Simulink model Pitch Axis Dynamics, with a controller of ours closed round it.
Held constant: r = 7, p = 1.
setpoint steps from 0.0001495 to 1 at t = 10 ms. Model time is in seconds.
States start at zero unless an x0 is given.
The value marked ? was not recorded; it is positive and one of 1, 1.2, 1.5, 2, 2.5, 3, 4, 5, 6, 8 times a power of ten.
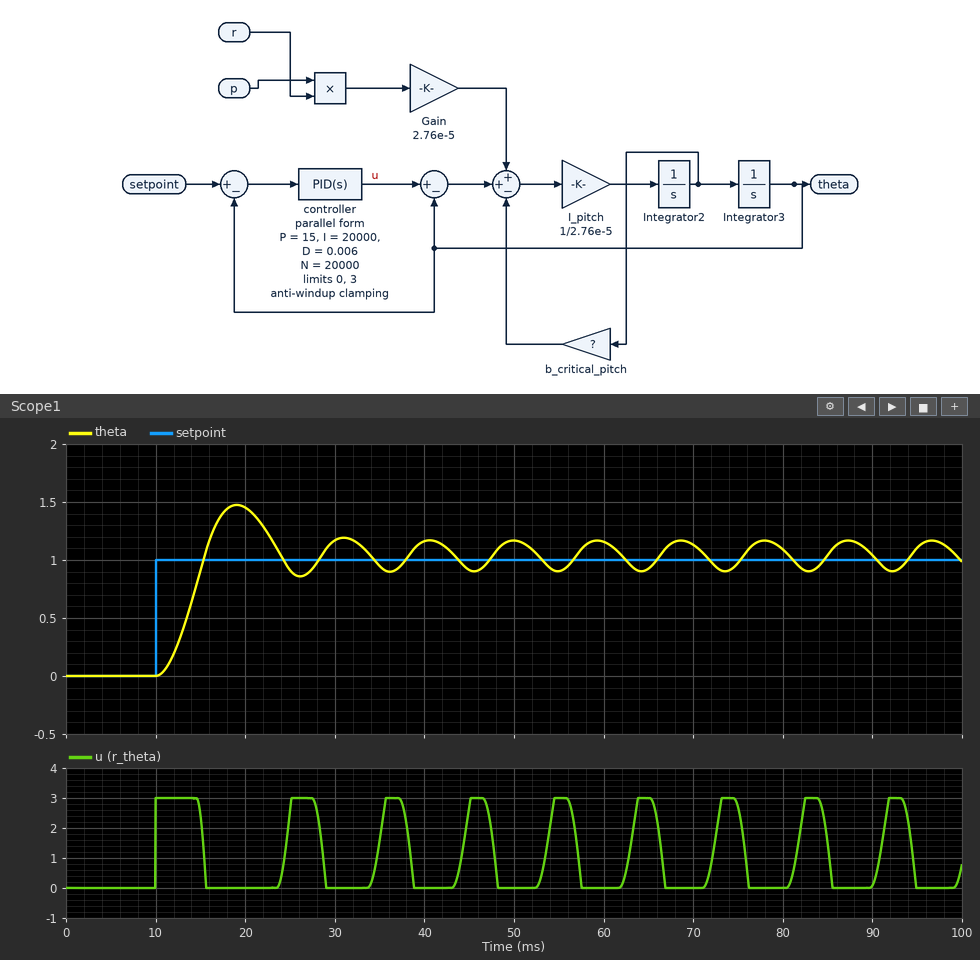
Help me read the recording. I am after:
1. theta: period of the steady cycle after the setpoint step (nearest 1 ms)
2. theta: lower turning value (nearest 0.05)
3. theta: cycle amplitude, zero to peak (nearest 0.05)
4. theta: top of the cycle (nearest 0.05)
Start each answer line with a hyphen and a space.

- 9 ms
- 0.90
- 0.15
- 1.15
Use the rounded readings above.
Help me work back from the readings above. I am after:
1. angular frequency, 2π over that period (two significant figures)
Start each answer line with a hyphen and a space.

- 0.70 rad/ms
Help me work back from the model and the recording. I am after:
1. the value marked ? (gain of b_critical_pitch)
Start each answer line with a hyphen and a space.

- 0.006
